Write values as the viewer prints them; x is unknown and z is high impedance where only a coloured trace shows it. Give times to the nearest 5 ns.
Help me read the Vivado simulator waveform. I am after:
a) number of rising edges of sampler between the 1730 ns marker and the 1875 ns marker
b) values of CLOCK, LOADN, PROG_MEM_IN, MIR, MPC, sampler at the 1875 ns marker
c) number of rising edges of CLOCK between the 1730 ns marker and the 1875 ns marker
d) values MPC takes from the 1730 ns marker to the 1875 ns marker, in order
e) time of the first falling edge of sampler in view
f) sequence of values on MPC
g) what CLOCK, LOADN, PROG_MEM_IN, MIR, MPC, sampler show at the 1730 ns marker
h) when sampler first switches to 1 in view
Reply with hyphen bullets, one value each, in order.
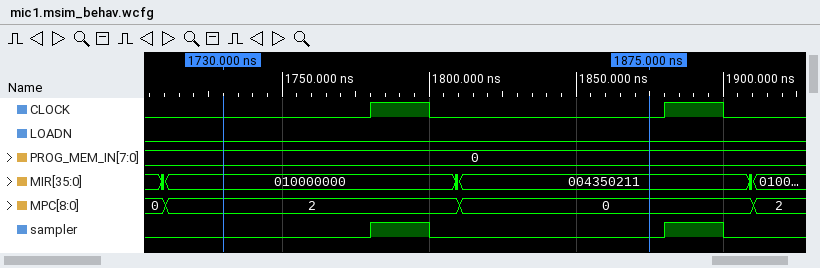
- 1
- CLOCK=0, LOADN=0, PROG_MEM_IN=0, MIR=004350211, MPC=0, sampler=0
- 1
- 2, 0
- 1800 ns
- 0, 2, 0, 2
- CLOCK=0, LOADN=0, PROG_MEM_IN=0, MIR=010000000, MPC=2, sampler=0
- 1780 ns
